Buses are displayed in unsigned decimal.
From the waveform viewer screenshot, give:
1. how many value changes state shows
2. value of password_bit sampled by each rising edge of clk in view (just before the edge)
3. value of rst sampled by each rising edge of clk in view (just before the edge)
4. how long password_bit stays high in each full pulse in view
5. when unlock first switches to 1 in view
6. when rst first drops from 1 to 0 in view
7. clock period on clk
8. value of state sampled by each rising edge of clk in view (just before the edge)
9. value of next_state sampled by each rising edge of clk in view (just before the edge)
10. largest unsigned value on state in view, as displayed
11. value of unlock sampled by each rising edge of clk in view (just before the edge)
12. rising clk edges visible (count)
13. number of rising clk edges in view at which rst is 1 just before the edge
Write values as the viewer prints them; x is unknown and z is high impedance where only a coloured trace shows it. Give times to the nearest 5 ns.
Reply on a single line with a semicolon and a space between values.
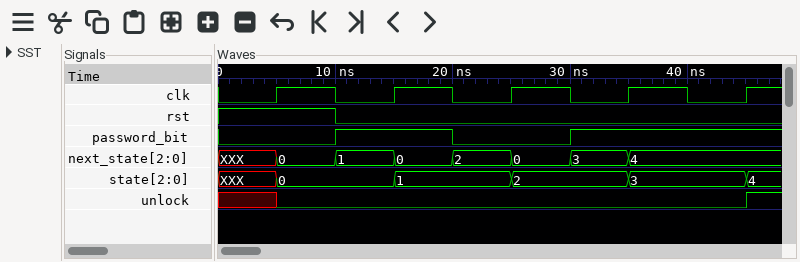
5; 0 1 0 1 1; 1 0 0 0 0; 10 ns; 45 ns; 10 ns; 10 ns; XXX, 0, 1, 2, 3; XXX, 1, 2, 3, 4; 4; x 0 0 0 0; 5; 1
